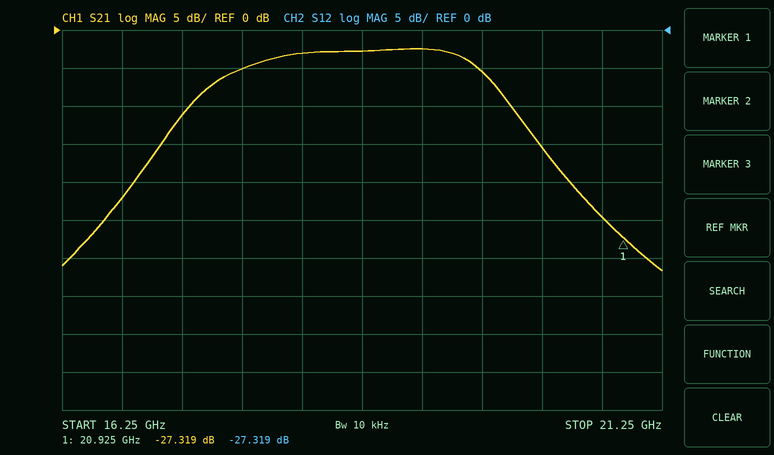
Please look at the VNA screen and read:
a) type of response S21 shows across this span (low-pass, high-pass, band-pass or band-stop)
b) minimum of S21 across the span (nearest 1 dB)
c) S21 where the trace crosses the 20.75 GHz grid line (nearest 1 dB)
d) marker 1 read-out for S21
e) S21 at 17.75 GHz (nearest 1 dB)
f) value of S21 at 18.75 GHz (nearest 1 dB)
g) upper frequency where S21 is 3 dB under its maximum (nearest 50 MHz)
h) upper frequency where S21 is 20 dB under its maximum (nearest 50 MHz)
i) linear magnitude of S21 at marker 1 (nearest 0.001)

band-pass
-32 dB
-25 dB
-27.319 dB
-5 dB
-3 dB
19.75 GHz
20.60 GHz
0.043
